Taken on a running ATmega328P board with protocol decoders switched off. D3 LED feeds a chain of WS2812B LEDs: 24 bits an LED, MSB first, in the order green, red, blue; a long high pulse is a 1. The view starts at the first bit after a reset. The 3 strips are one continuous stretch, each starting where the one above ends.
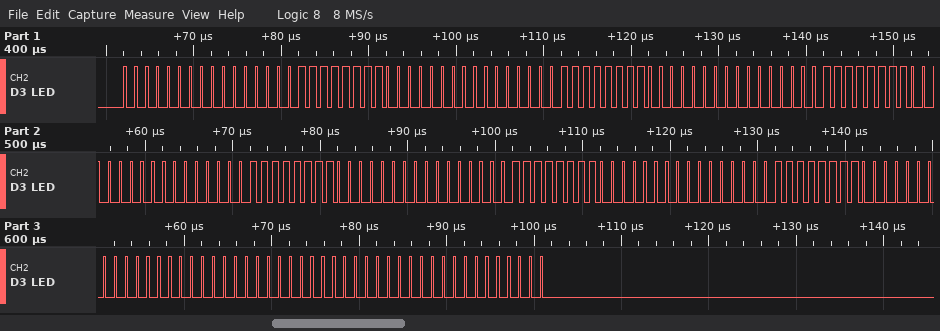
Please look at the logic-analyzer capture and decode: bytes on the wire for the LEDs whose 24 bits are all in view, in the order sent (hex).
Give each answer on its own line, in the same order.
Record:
00 00 FF 00 00 FF 00 00 FF 00 00 FF 00 00 FF 00 00 FF 00 00 00 00 00 00
